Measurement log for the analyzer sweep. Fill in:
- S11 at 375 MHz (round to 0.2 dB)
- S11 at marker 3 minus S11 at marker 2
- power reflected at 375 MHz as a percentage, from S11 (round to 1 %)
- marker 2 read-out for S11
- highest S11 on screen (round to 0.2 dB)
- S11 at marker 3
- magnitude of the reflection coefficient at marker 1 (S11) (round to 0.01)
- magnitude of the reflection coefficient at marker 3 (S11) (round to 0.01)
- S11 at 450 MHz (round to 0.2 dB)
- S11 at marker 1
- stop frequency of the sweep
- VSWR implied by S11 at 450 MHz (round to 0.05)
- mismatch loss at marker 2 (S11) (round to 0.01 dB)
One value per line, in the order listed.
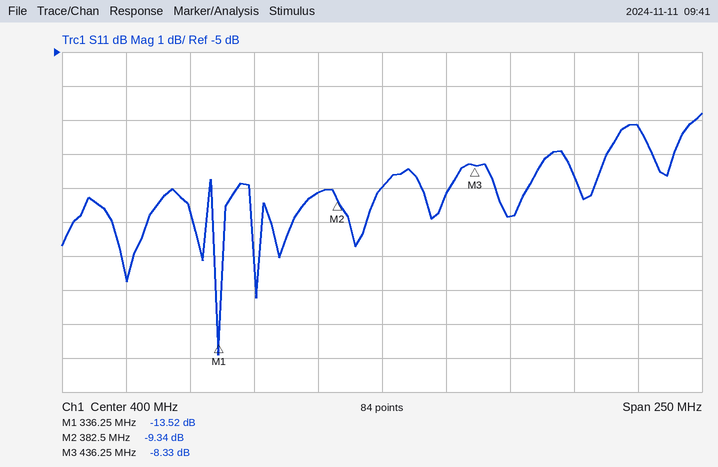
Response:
-9.2 dB
1.01 dB
12 %
-9.34 dB
-6.8 dB
-8.33 dB
0.21
0.38
-9.8 dB
-13.52 dB
525 MHz
1.95
0.54 dB
